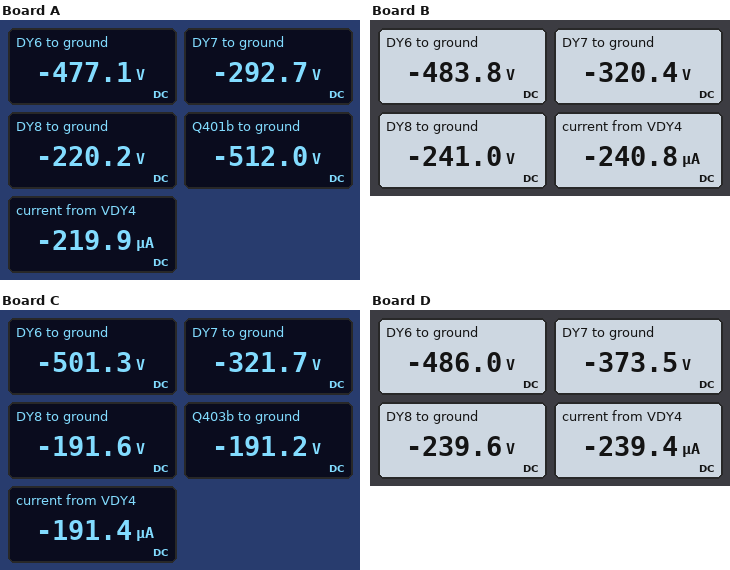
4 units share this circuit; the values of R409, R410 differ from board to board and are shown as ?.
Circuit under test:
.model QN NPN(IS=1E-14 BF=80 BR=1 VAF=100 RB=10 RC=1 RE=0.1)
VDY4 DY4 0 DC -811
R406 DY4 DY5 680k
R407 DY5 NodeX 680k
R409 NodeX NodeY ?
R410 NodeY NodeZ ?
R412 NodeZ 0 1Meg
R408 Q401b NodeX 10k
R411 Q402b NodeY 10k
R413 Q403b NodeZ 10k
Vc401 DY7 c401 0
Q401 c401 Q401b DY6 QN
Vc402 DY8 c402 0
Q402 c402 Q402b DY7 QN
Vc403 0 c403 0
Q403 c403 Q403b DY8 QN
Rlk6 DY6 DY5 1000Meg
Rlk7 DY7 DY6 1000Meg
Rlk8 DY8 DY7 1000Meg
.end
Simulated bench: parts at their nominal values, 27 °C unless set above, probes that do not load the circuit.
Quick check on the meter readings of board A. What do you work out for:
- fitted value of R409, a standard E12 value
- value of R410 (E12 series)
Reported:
1 MΩ
330 kΩ
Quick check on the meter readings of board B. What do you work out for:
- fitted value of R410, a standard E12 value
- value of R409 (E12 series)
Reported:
330 kΩ
680 kΩ
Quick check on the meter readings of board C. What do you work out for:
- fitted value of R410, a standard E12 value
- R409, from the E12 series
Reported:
680 kΩ
1.2 MΩ
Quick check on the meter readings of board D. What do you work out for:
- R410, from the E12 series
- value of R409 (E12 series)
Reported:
560 kΩ
470 kΩ
